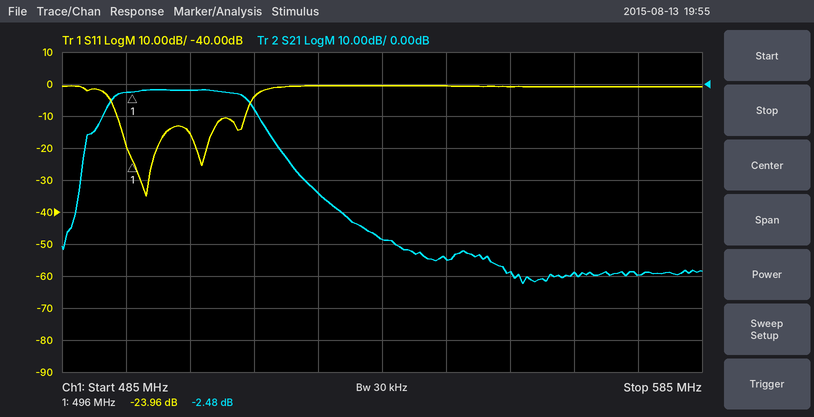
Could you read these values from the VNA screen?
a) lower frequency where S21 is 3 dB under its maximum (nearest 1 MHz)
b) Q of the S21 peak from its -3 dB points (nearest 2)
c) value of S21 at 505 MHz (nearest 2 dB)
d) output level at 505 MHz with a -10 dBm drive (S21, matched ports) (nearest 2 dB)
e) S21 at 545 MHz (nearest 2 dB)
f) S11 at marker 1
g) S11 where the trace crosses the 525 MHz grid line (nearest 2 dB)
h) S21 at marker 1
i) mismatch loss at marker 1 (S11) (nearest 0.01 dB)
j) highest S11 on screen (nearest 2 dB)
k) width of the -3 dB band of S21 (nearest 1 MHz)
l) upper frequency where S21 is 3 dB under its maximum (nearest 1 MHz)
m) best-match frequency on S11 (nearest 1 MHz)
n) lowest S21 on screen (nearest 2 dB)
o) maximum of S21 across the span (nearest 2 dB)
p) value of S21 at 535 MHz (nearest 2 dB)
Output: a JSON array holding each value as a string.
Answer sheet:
["493 MHz", "24", "-2 dB", "-12 dBm", "-54 dB", "-23.96 dB", "0 dB", "-2.48 dB", "0.02 dB", "0 dB", "21 MHz", "514 MHz", "498 MHz", "-62 dB", "-2 dB", "-48 dB"]
